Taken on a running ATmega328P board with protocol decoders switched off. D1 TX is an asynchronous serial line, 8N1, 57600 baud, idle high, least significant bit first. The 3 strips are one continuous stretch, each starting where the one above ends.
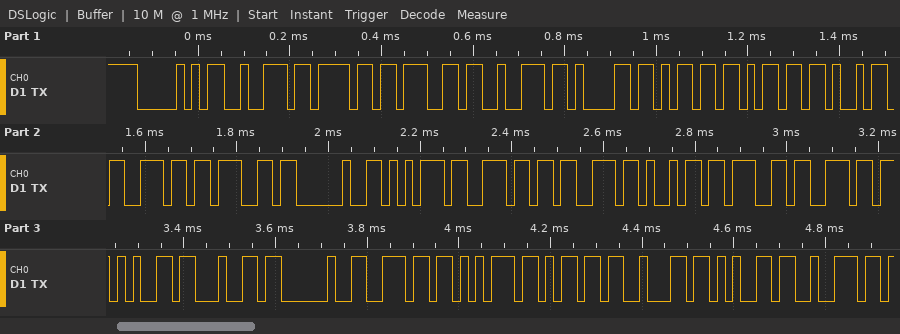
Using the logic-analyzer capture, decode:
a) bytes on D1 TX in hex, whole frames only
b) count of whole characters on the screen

50 72 6F 67 72 61 6D 6D 69 6E 67 20 75 6E 73 69 67 6E 65 64 20 6E 75 6D 62 65 72
27
